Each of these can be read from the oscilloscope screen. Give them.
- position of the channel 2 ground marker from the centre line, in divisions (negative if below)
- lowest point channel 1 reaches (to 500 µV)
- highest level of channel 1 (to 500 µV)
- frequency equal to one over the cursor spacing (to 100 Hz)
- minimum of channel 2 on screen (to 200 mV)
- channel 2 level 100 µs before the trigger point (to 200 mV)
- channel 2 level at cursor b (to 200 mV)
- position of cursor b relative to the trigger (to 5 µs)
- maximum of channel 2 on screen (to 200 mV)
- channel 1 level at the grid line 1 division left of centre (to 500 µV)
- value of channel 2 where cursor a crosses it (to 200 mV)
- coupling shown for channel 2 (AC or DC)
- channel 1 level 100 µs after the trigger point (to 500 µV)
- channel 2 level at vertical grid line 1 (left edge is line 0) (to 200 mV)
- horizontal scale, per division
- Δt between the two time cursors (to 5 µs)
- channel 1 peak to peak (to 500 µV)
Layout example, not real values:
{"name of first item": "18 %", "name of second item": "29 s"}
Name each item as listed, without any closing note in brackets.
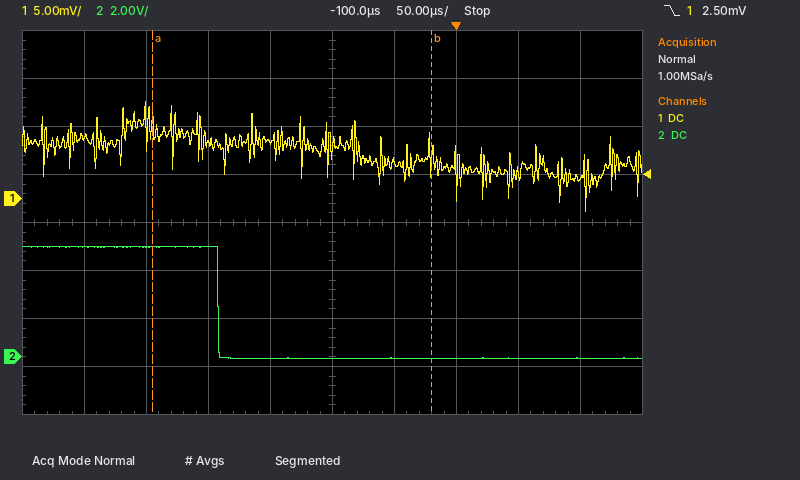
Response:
{"position of the channel 2 ground marker from the centre line, in divisions": "-2.8 div", "lowest point channel 1 reaches": "-1.5 mV", "highest level of channel 1": "10.0 mV", "frequency equal to one over the cursor spacing": "4.4 kHz", "minimum of channel 2 on screen": "0.0 V", "channel 2 level 100 µs before the trigger point": "0.0 V", "channel 2 level at cursor b": "0.0 V", "position of cursor b relative to the trigger": "-20 µs", "maximum of channel 2 on screen": "4.6 V", "channel 1 level at the grid line 1 division left of centre": "6.0 mV", "value of channel 2 where cursor a crosses it": "4.6 V", "coupling shown for channel 2": "DC", "channel 1 level 100 µs after the trigger point": "2.0 mV", "channel 2 level at vertical grid line 1 (left edge is line 0)": "4.6 V", "horizontal scale, per division": "50 µs", "Δt between the two time cursors": "225 µs", "channel 1 peak to peak": "11.5 mV"}
